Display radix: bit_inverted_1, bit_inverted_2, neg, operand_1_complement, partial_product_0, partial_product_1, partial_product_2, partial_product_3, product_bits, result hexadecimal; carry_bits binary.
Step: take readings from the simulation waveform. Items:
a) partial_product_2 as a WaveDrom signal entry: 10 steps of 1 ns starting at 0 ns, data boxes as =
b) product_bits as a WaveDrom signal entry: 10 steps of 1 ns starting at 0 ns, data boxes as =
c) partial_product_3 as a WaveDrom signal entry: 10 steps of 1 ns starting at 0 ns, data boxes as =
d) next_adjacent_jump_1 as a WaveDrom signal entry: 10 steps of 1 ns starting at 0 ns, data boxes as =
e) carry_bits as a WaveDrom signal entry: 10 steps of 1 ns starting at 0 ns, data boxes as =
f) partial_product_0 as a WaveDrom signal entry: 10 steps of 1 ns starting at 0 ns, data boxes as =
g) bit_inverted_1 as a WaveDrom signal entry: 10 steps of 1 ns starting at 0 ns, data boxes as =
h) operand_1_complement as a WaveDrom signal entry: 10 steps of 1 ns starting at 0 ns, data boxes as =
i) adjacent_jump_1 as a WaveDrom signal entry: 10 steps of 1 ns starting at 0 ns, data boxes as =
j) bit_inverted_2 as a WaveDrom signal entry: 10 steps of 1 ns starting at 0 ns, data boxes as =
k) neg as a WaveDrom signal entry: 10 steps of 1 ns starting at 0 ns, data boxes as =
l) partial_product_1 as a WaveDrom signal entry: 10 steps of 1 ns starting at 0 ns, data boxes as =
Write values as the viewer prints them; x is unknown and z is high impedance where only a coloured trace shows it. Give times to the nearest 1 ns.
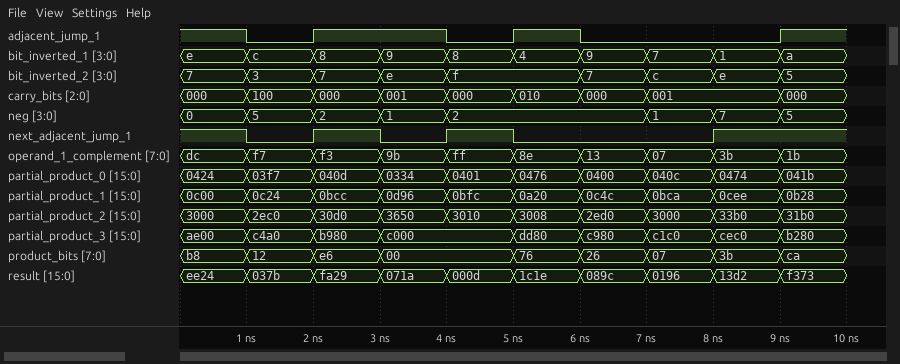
{name: 'partial_product_2', wave: '==========', data: '3000 2ec0 30d0 3650 3010 3008 2ed0 3000 33b0 31b0'}
{name: 'product_bits', wave: '====.=====', data: 'b8 12 e6 00 76 26 07 3b ca'}
{name: 'partial_product_3', wave: '====.=====', data: 'ae00 c4a0 b980 c000 dd80 c980 c1c0 cec0 b280'}
{name: 'next_adjacent_jump_1', wave: '101010..1.'}
{name: 'carry_bits', wave: '========.=', data: '000 100 000 001 000 010 000 001 000'}
{name: 'partial_product_0', wave: '==========', data: '0424 03f7 040d 0334 0401 0476 0400 040c 0474 041b'}
{name: 'bit_inverted_1', wave: '==========', data: 'e c 8 9 8 4 9 7 1 a'}
{name: 'operand_1_complement', wave: '==========', data: 'dc f7 f3 9b ff 8e 13 07 3b 1b'}
{name: 'adjacent_jump_1', wave: '101.010..1'}
{name: 'bit_inverted_2', wave: '=====.====', data: '7 3 7 e f 7 c e 5'}
{name: 'neg', wave: '=====..===', data: '0 5 2 1 2 1 7 5'}
{name: 'partial_product_1', wave: '==========', data: '0c00 0c24 0bcc 0d96 0bfc 0a20 0c4c 0bca 0cee 0b28'}
